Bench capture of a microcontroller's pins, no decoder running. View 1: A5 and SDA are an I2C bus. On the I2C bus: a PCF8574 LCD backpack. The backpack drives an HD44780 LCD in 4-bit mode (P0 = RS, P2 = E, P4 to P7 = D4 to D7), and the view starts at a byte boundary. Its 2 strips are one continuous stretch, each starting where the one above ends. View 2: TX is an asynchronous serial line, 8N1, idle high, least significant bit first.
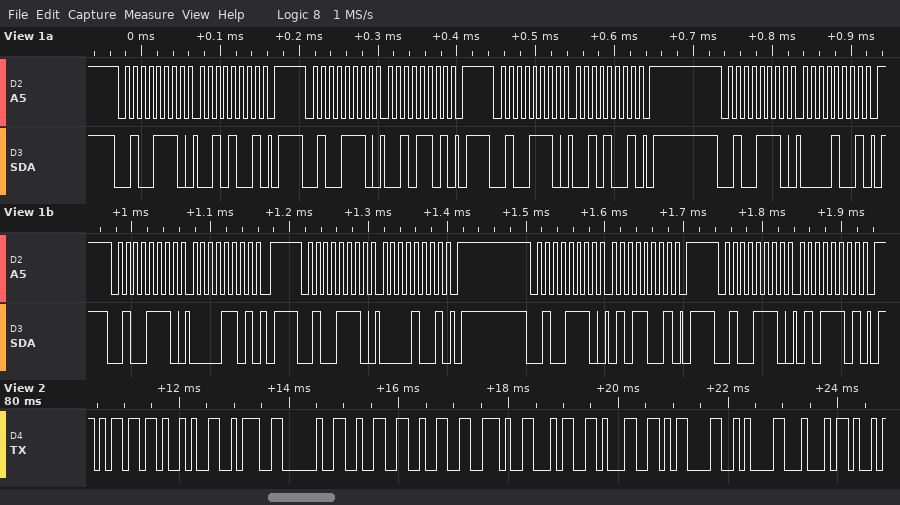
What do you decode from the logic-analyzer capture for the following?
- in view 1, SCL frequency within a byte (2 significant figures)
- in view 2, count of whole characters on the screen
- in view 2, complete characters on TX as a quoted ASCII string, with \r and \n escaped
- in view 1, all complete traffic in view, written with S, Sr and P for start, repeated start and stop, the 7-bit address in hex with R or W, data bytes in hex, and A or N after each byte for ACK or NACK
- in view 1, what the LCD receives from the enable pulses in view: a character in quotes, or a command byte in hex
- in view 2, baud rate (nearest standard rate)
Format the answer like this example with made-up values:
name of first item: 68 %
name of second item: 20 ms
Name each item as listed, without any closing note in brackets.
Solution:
in view 1, SCL frequency within a byte: 100 kHz
in view 2, count of whole characters on the screen: 12
in view 2, complete characters on TX as a quoted ASCII string, with \r and \n escaped: "m): 22.41\r\nD"
in view 1, all complete traffic in view, written with S, Sr and P for start, repeated start and stop, the 7-bit address in hex with R or W, data bytes in hex, and A or N after each byte for ACK or NACK: S 27W A 29 A P S 27W A 2D A P S 27W A 29 A P S 27W A 09 A P S 27W A 0D A P S 27W A 09 A P S 27W A 59 A P S 27W A 5D A P
in view 1, what the LCD receives from the enable pulses in view: a character in quotes, or a command byte in hex: ' '
in view 2, baud rate: 9600 baud
